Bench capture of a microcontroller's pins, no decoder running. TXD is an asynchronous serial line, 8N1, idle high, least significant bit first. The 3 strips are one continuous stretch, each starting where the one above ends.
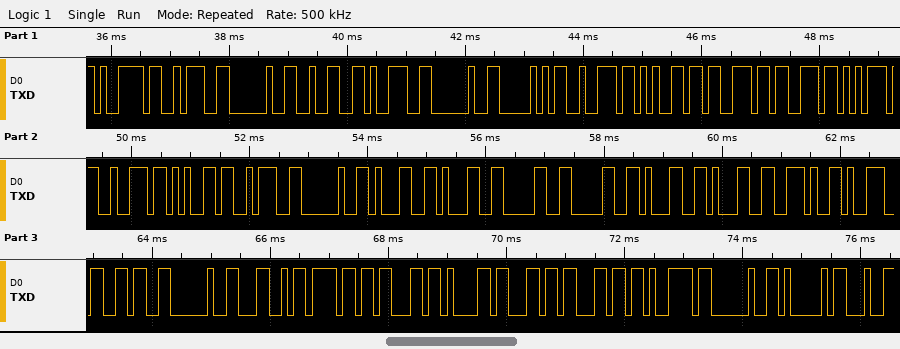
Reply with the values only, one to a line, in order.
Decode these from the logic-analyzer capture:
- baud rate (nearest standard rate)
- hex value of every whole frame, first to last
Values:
9600 baud
79 3A 20 32 39 20 50 72 65 73 73 75 72 65 3A 20 31 31 30 30 31 31 2E 39 36 20 4C 6F 63 61 6C 6C 79 20 41
